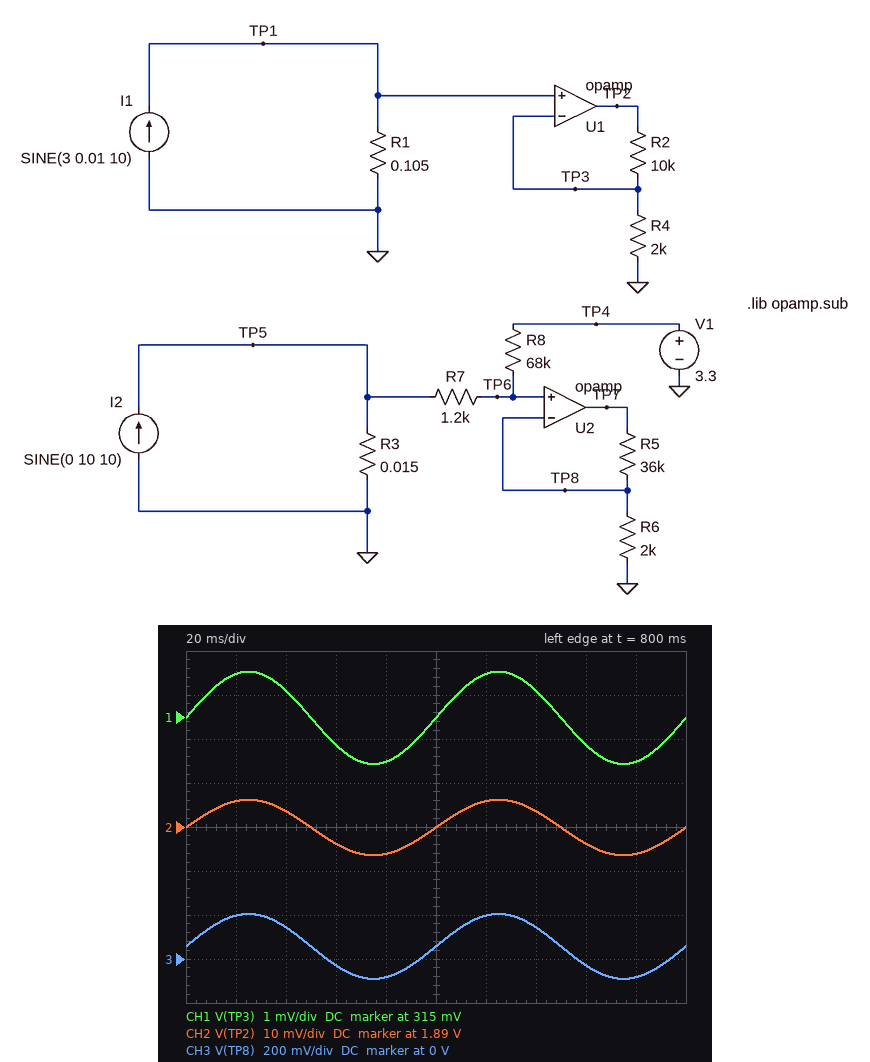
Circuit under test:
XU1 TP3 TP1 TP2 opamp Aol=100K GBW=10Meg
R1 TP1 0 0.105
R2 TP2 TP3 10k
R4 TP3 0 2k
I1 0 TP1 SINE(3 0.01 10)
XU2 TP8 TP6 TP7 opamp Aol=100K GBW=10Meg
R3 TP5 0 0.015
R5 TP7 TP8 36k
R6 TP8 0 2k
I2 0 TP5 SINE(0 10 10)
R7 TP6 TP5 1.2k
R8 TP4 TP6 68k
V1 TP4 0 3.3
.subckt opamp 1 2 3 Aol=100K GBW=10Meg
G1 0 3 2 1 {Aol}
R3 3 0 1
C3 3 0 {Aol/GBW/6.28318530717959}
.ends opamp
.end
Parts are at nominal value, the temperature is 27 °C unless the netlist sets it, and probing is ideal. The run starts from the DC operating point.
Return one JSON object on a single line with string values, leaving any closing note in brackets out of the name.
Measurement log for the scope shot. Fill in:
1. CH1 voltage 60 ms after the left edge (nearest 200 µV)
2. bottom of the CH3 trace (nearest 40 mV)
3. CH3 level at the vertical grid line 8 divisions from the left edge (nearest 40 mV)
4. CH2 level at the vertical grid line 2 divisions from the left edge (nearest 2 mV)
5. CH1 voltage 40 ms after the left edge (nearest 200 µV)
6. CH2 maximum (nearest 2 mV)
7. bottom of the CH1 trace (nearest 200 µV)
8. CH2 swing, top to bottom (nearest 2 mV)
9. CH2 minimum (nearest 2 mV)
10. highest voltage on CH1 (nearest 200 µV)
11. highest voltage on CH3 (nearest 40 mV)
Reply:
{"CH1 voltage 60 ms after the left edge": "314.4 mV", "bottom of the CH3 trace": "-80 mV", "CH3 level at the vertical grid line 8 divisions from the left edge": "-40 mV", "CH2 level at the vertical grid line 2 divisions from the left edge": "1.894 V", "CH1 voltage 40 ms after the left edge": "315.6 mV", "CH2 maximum": "1.896 V", "bottom of the CH1 trace": "314.0 mV", "CH2 swing, top to bottom": "12 mV", "CH2 minimum": "1.884 V", "highest voltage on CH1": "316.0 mV", "highest voltage on CH3": "200 mV"}
